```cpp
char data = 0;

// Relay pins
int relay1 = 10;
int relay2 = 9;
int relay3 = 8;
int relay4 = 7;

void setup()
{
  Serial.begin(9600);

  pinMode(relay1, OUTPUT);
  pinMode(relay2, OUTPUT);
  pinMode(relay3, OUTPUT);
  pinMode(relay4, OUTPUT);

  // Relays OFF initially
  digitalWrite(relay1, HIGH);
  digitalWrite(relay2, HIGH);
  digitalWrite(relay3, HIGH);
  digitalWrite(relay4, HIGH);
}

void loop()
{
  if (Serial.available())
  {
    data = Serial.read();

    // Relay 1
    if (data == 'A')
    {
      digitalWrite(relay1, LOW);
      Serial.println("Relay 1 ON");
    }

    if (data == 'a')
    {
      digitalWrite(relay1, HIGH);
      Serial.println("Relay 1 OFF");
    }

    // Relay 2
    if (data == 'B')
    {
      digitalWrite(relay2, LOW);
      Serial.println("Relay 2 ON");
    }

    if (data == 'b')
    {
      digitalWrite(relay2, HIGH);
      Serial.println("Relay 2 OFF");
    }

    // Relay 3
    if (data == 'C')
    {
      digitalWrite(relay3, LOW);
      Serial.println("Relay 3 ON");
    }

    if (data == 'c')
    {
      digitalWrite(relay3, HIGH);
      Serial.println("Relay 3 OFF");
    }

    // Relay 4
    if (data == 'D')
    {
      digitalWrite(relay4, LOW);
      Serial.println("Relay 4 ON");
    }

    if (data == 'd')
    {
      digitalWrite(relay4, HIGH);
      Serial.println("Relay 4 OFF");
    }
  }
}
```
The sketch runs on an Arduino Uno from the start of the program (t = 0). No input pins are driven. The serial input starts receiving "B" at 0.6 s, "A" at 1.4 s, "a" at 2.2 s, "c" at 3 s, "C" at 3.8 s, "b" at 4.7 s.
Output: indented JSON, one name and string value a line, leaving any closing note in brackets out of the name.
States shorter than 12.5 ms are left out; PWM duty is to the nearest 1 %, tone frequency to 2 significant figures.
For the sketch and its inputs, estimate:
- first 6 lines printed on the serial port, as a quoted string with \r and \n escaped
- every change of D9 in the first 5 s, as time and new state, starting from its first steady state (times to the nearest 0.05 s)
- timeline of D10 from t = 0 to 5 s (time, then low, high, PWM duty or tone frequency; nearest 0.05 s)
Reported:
{
  "first 6 lines printed on the serial port, as a quoted string with \\r and \\n escaped": "\"Relay 2 ON\\r\\nRelay 1 ON\\r\\nRelay 1 OFF\\r\\nRelay 3 OFF\\r\\nRelay 3 ON\\r\\nRelay 2 OFF\\r\\n\"",
  "every change of D9 in the first 5 s, as time and new state, starting from its first steady state": "0 s high; 0.6 s low; 4.7 s high",
  "timeline of D10 from t = 0 to 5 s": "0 s high; 1.4 s low; 2.2 s high"
}
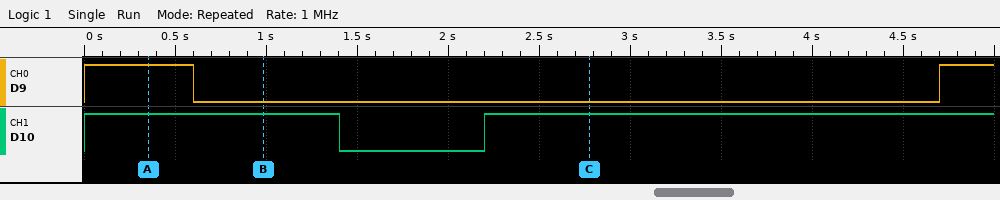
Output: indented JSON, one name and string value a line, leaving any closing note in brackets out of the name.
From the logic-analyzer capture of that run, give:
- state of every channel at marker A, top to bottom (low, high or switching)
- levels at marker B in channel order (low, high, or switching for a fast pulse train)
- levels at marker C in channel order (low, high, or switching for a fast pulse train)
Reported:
{
  "state of every channel at marker A, top to bottom": "D9 high, D10 high",
  "levels at marker B in channel order": "D9 low, D10 high",
  "levels at marker C in channel order": "D9 low, D10 high"
}
